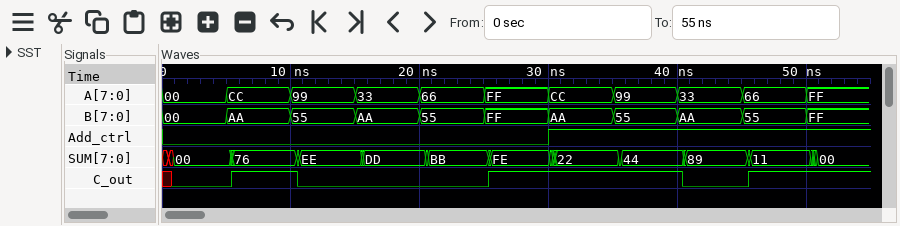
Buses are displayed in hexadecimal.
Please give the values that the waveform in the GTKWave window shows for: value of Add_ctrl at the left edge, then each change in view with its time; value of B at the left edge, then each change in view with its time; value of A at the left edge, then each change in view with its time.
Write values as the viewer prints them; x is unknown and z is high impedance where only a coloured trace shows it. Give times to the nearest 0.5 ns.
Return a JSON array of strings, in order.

["0, 1 at 30 ns", "00, AA at 5 ns, 55 at 10 ns, AA at 15 ns, 55 at 20 ns, FF at 25 ns, AA at 30 ns, 55 at 35 ns, AA at 40 ns, 55 at 45 ns, FF at 50 ns", "00, CC at 5 ns, 99 at 10 ns, 33 at 15 ns, 66 at 20 ns, FF at 25 ns, CC at 30 ns, 99 at 35 ns, 33 at 40 ns, 66 at 45 ns, FF at 50 ns"]
